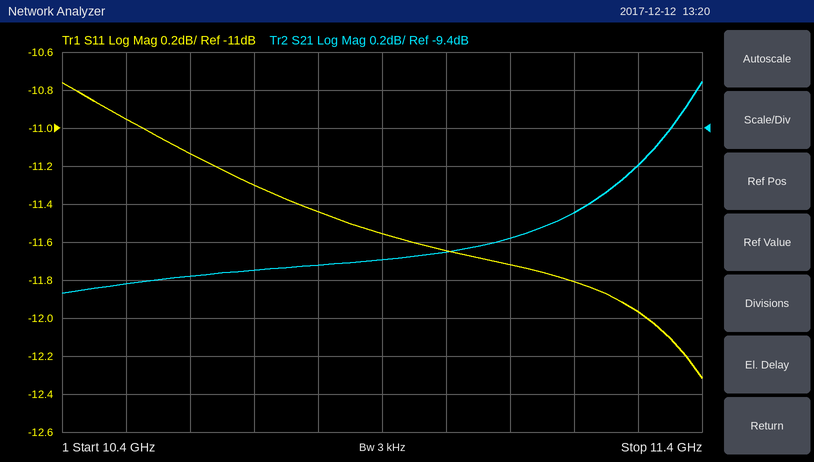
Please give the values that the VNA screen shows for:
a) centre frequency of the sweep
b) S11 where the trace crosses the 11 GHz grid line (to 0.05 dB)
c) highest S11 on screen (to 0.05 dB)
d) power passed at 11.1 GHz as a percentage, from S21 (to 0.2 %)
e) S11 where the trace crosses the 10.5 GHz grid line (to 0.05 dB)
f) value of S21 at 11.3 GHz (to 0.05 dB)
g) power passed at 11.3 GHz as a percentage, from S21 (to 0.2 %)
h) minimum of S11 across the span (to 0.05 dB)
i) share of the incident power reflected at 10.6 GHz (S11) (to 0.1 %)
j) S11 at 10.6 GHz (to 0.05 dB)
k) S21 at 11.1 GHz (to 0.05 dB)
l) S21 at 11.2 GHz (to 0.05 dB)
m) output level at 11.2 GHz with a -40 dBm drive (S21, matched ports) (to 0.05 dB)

10.9 GHz
-11.65 dB
-10.75 dB
10.0 %
-10.95 dB
-9.60 dB
11.0 %
-12.30 dB
7.7 %
-11.15 dB
-10.00 dB
-9.85 dB
-49.85 dBm
